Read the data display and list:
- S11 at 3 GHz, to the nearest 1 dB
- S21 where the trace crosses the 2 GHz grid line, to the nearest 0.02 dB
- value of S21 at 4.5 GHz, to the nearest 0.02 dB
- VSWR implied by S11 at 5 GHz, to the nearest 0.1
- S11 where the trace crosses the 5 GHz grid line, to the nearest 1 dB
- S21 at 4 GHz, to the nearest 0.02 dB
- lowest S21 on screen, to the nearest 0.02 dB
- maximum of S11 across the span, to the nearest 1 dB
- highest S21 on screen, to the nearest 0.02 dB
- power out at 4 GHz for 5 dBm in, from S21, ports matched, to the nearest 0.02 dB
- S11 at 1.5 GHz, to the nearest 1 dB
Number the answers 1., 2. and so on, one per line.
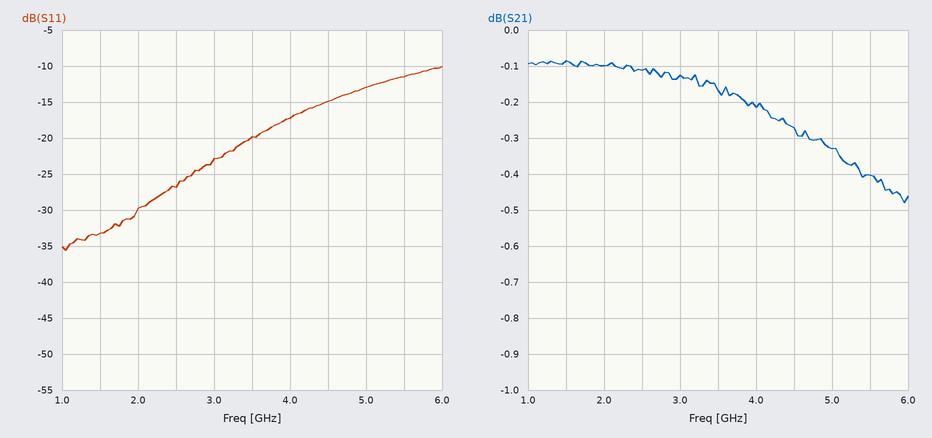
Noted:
1. -23 dB
2. -0.10 dB
3. -0.28 dB
4. 1.6
5. -13 dB
6. -0.22 dB
7. -0.48 dB
8. -10 dB
9. -0.08 dB
10. 4.78 dBm
11. -33 dB
